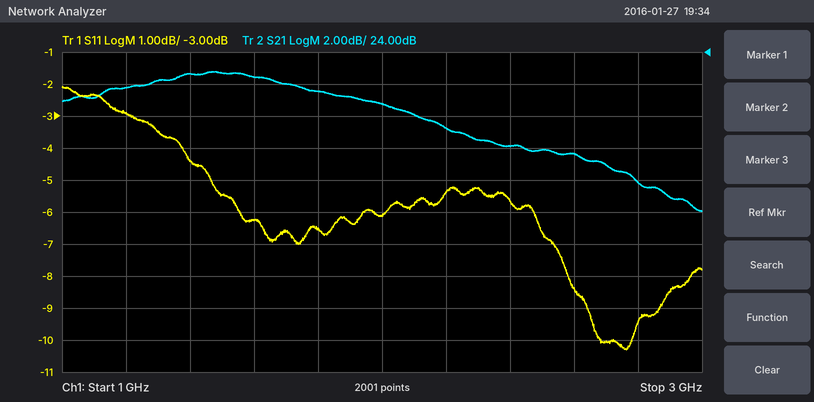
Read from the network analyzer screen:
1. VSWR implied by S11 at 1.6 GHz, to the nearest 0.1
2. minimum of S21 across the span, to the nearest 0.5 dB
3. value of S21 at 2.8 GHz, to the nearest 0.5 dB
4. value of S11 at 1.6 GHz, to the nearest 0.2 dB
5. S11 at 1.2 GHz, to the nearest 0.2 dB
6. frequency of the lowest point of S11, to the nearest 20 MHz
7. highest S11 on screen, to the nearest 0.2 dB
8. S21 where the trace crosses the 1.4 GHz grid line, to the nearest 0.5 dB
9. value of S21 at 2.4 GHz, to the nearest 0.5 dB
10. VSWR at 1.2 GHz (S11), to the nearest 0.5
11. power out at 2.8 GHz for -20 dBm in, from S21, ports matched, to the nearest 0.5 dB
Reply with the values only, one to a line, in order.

2.9
14.0 dB
16.0 dB
-6.2 dB
-3.0 dB
2.76 GHz
-2.0 dB
22.5 dB
18.0 dB
6.0
-4.0 dBm
